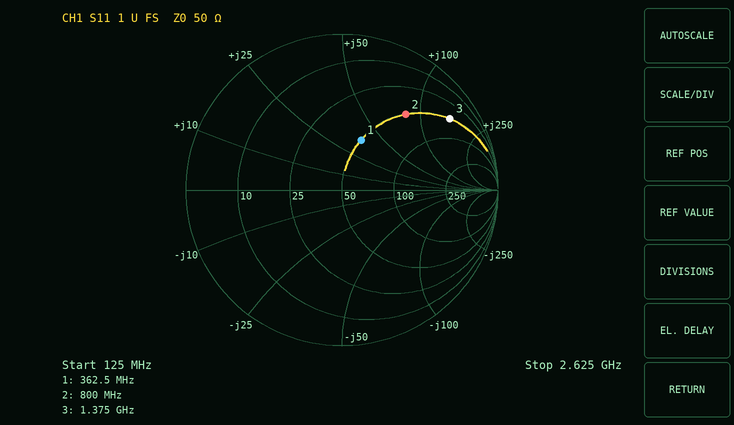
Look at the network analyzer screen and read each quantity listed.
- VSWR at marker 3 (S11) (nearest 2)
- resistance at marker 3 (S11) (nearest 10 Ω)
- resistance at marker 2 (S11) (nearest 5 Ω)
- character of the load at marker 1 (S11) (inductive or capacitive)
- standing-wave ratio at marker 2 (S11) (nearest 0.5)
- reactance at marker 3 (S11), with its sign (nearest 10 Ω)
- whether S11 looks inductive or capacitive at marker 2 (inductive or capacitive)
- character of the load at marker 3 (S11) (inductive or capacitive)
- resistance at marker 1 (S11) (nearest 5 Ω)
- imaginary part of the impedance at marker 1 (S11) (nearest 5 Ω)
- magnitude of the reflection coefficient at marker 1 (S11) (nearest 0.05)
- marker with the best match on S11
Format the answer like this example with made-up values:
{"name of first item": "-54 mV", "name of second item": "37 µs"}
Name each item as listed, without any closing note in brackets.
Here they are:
{"VSWR at marker 3 (S11)": "10", "resistance at marker 3 (S11)": "50 Ω", "resistance at marker 2 (S11)": "50 Ω", "character of the load at marker 1 (S11)": "inductive", "standing-wave ratio at marker 2 (S11)": "4.5", "reactance at marker 3 (S11), with its sign": "+150 Ω", "whether S11 looks inductive or capacitive at marker 2": "inductive", "character of the load at marker 3 (S11)": "inductive", "resistance at marker 1 (S11)": "50 Ω", "imaginary part of the impedance at marker 1 (S11)": "+35 Ω", "magnitude of the reflection coefficient at marker 1 (S11)": "0.35", "marker with the best match on S11": "marker 1"}
